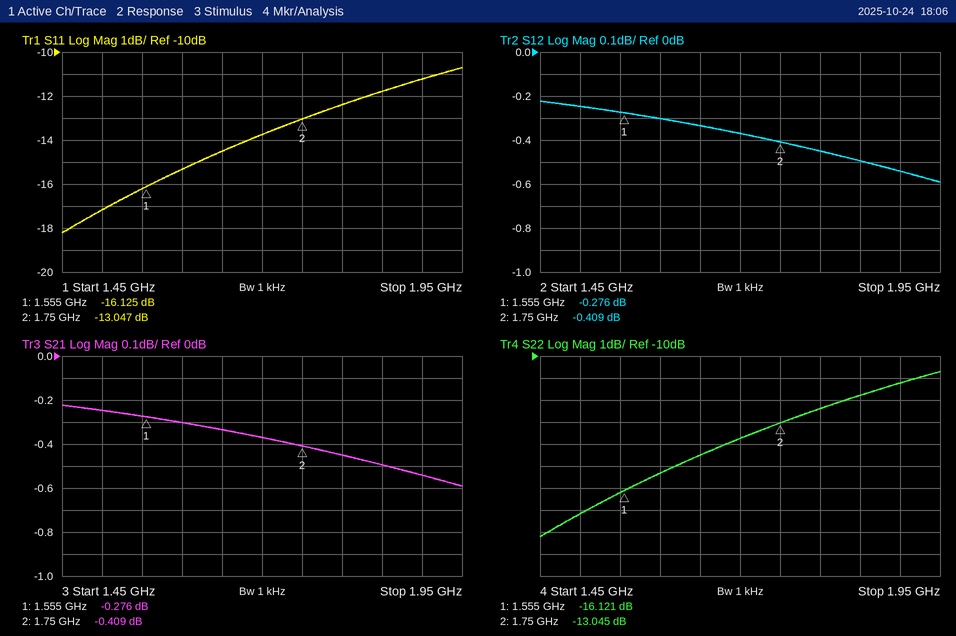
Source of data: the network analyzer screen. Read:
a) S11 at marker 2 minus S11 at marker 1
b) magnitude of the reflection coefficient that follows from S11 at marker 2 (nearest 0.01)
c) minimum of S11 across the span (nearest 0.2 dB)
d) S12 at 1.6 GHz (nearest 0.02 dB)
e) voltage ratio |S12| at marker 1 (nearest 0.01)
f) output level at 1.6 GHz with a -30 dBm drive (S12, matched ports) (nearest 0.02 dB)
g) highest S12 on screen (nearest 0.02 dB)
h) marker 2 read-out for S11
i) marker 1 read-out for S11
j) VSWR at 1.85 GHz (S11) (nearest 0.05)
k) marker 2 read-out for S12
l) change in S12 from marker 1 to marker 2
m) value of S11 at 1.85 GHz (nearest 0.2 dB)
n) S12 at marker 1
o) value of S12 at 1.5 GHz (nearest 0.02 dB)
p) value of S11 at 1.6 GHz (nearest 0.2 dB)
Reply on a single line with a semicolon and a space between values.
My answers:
3.078 dB; 0.22; -18.2 dB; -0.30 dB; 0.97; -30.30 dBm; -0.22 dB; -13.047 dB; -16.125 dB; 1.70; -0.409 dB; -0.133 dB; -11.8 dB; -0.276 dB; -0.24 dB; -15.4 dB
